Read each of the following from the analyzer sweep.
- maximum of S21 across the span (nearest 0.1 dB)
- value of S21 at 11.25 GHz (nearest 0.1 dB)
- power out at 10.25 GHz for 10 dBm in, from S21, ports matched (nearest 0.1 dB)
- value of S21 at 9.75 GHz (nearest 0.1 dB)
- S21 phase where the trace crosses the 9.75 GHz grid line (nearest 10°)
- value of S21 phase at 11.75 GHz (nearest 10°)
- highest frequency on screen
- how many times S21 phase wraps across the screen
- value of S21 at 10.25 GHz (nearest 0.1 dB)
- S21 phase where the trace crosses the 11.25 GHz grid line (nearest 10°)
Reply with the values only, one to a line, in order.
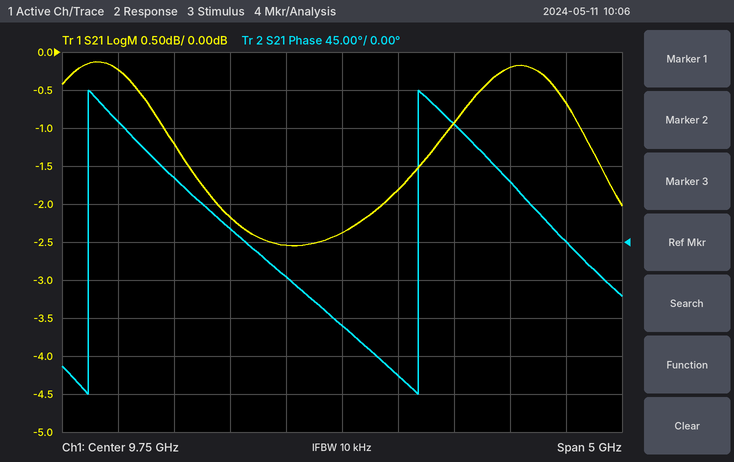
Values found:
-0.1 dB
-0.2 dB
8.2 dBm
-2.4 dB
-100°
0°
12.25 GHz
2
-1.8 dB
70°
